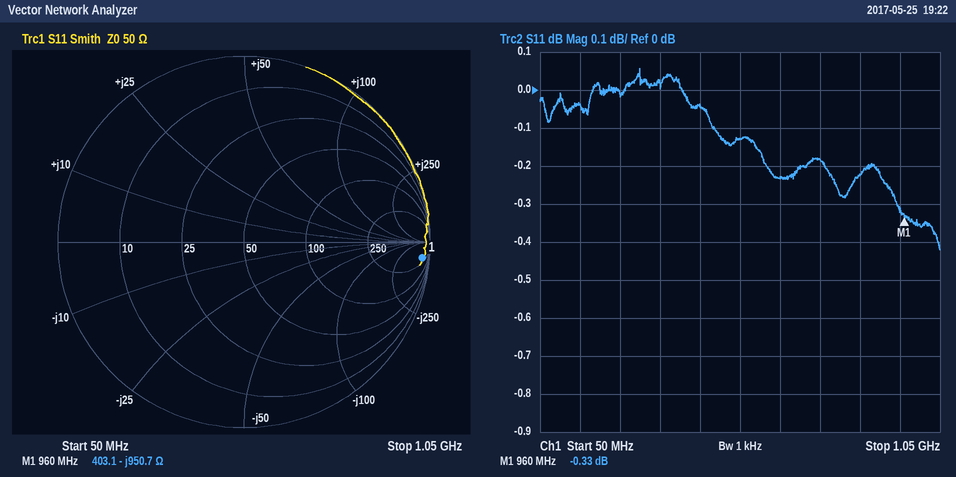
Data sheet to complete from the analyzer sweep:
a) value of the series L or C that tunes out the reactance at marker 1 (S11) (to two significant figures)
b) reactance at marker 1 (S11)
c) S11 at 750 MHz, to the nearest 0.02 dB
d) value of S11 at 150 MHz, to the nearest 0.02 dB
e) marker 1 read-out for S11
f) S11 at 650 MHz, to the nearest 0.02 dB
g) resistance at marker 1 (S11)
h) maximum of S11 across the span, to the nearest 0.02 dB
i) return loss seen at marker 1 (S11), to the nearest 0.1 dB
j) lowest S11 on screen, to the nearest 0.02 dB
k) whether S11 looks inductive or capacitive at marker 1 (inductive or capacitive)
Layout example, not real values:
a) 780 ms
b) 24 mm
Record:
a) 160 nH
b) -950.7 Ω
c) -0.18 dB
d) -0.04 dB
e) -0.33 dB
f) -0.24 dB
g) 403.1 Ω
h) 0.06 dB
i) 0.3 dB
j) -0.42 dB
k) capacitive
